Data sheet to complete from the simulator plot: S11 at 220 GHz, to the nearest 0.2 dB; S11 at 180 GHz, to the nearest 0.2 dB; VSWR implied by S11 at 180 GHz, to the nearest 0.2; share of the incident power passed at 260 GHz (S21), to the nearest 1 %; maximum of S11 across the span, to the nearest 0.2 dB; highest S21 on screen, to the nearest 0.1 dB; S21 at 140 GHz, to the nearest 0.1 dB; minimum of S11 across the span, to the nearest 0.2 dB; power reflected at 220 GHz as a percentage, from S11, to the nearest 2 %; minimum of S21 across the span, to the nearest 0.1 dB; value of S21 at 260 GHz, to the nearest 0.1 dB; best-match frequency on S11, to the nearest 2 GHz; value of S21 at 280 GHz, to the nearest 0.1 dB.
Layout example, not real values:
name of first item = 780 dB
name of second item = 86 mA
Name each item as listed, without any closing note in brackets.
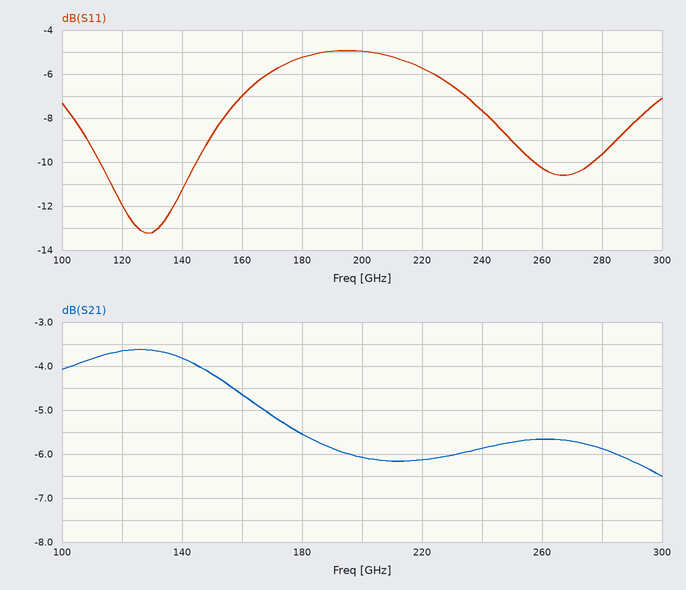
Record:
S11 at 220 GHz, to the nearest 0.2 dB = -5.8 dB
S11 at 180 GHz, to the nearest 0.2 dB = -5.2 dB
VSWR implied by S11 at 180 GHz, to the nearest 0.2 = 3.4
share of the incident power passed at 260 GHz (S21), to the nearest 1 % = 27 %
maximum of S11 across the span, to the nearest 0.2 dB = -5.0 dB
highest S21 on screen, to the nearest 0.1 dB = -3.6 dB
S21 at 140 GHz, to the nearest 0.1 dB = -3.8 dB
minimum of S11 across the span, to the nearest 0.2 dB = -13.2 dB
power reflected at 220 GHz as a percentage, from S11, to the nearest 2 % = 26 %
minimum of S21 across the span, to the nearest 0.1 dB = -6.5 dB
value of S21 at 260 GHz, to the nearest 0.1 dB = -5.7 dB
best-match frequency on S11, to the nearest 2 GHz = 128 GHz
value of S21 at 280 GHz, to the nearest 0.1 dB = -5.9 dB
